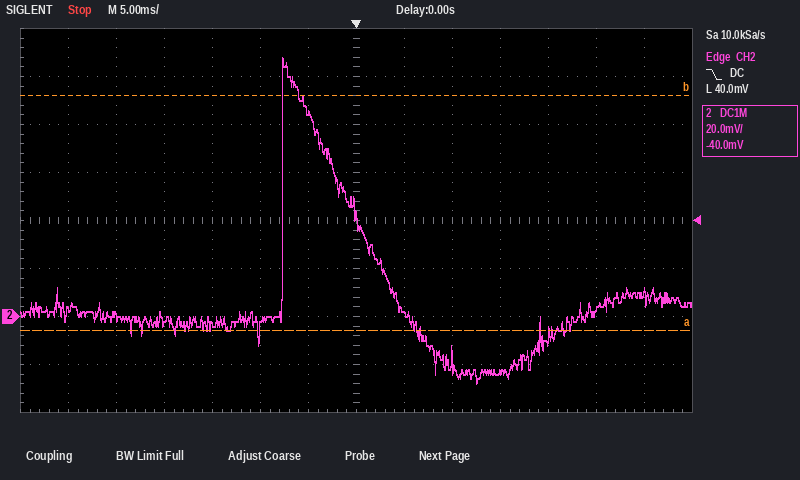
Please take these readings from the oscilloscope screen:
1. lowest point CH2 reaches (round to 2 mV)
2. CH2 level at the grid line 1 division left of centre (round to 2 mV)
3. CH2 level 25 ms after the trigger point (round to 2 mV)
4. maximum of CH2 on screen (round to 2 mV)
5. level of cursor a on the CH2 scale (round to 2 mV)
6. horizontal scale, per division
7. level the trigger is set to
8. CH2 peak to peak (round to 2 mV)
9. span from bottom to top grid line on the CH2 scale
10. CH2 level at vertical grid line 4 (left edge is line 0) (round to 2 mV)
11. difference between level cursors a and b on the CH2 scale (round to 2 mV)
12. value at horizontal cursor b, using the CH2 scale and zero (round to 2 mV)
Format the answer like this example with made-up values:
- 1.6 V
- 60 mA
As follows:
- -28 mV
- 86 mV
- 2 mV
- 108 mV
- -6 mV
- 5 ms
- 40.0 mV
- 136 mV
- 160 mV
- -4 mV
- 98 mV
- 92 mV
